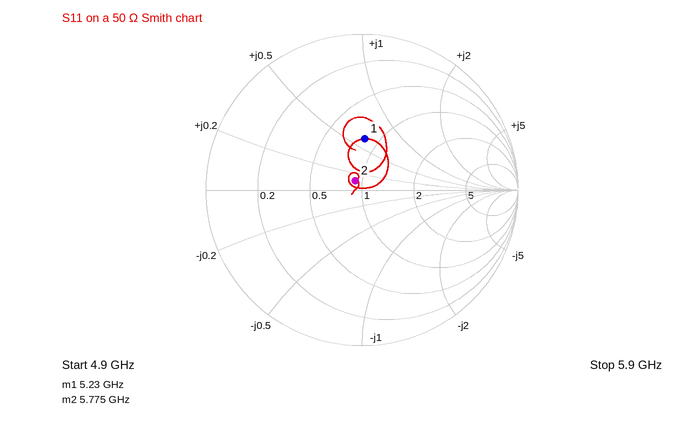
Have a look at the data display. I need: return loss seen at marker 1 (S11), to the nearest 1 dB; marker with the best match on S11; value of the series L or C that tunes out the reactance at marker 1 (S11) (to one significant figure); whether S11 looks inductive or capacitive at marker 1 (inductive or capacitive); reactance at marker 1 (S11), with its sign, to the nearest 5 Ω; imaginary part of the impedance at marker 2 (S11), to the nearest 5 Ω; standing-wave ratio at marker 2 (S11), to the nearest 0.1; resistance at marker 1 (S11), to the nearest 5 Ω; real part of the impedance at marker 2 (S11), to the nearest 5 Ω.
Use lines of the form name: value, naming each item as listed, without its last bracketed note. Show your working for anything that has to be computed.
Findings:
return loss seen at marker 1 (S11), to the nearest 1 dB: 10 dB
marker with the best match on S11: marker 2
value of the series L or C that tunes out the reactance at marker 1 (S11): C = 1/(2π × 5.23 GHz × 30 Ω) ≈ 1.0 pF
whether S11 looks inductive or capacitive at marker 1: inductive
reactance at marker 1 (S11), with its sign, to the nearest 5 Ω: +30 Ω
imaginary part of the impedance at marker 2 (S11), to the nearest 5 Ω: +5 Ω
standing-wave ratio at marker 2 (S11), to the nearest 0.1: 1.2
resistance at marker 1 (S11), to the nearest 5 Ω: 40 Ω
real part of the impedance at marker 2 (S11), to the nearest 5 Ω: 45 Ω
